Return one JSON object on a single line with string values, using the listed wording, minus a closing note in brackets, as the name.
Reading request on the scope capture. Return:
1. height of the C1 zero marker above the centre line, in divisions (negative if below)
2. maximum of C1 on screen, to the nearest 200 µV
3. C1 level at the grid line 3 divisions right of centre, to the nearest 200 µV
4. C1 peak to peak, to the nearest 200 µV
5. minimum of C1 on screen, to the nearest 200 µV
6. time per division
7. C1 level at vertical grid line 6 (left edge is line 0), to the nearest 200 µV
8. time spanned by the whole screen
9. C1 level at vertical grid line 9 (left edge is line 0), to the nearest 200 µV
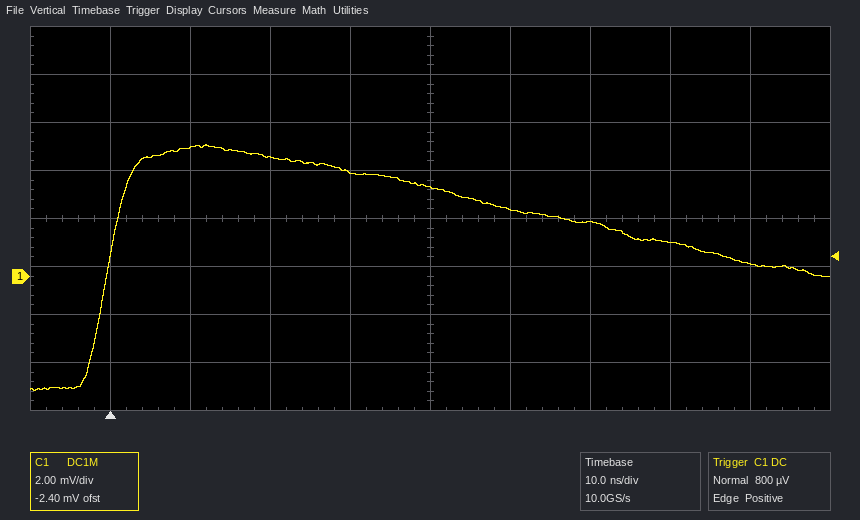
{"height of the C1 zero marker above the centre line, in divisions": "-1.2 div", "maximum of C1 on screen, to the nearest 200 µV": "5.4 mV", "C1 level at the grid line 3 divisions right of centre, to the nearest 200 µV": "1.4 mV", "C1 peak to peak, to the nearest 200 µV": "10.2 mV", "minimum of C1 on screen, to the nearest 200 µV": "-4.8 mV", "time per division": "10 ns", "C1 level at vertical grid line 6 (left edge is line 0), to the nearest 200 µV": "2.8 mV", "time spanned by the whole screen": "100 ns", "C1 level at vertical grid line 9 (left edge is line 0), to the nearest 200 µV": "600 µV"}
